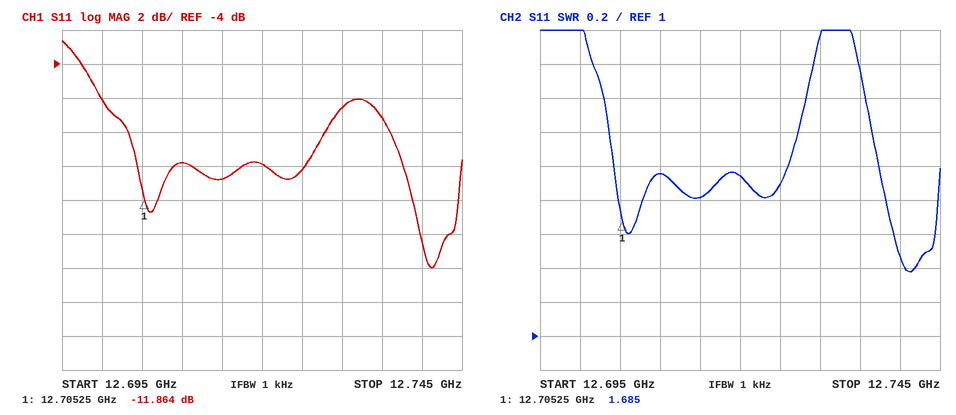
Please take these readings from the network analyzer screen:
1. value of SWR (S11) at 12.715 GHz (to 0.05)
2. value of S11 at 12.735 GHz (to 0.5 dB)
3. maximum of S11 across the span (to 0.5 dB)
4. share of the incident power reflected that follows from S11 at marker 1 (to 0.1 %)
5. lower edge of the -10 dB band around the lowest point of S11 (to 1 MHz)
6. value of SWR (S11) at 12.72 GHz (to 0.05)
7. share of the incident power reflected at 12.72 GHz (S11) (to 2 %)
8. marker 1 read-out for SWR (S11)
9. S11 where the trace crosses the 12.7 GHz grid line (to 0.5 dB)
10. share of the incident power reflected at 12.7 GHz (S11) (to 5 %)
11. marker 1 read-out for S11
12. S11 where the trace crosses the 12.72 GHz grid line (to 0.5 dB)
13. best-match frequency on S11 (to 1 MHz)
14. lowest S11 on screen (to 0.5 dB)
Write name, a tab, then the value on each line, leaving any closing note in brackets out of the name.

value of SWR (S11) at 12.715 GHz	1.80
value of S11 at 12.735 GHz	-7.0 dB
maximum of S11 across the span	-2.5 dB
share of the incident power reflected that follows from S11 at marker 1	6.5 %
lower edge of the -10 dB band around the lowest point of S11	12.738 GHz
value of SWR (S11) at 12.72 GHz	1.95
share of the incident power reflected at 12.72 GHz (S11)	10 %
marker 1 read-out for SWR	1.685
S11 where the trace crosses the 12.7 GHz grid line	-6.0 dB
share of the incident power reflected at 12.7 GHz (S11)	25 %
marker 1 read-out for S11	-11.864 dB
S11 where the trace crosses the 12.72 GHz grid line	-10.0 dB
best-match frequency on S11	12.741 GHz
lowest S11 on screen	-16.0 dB
